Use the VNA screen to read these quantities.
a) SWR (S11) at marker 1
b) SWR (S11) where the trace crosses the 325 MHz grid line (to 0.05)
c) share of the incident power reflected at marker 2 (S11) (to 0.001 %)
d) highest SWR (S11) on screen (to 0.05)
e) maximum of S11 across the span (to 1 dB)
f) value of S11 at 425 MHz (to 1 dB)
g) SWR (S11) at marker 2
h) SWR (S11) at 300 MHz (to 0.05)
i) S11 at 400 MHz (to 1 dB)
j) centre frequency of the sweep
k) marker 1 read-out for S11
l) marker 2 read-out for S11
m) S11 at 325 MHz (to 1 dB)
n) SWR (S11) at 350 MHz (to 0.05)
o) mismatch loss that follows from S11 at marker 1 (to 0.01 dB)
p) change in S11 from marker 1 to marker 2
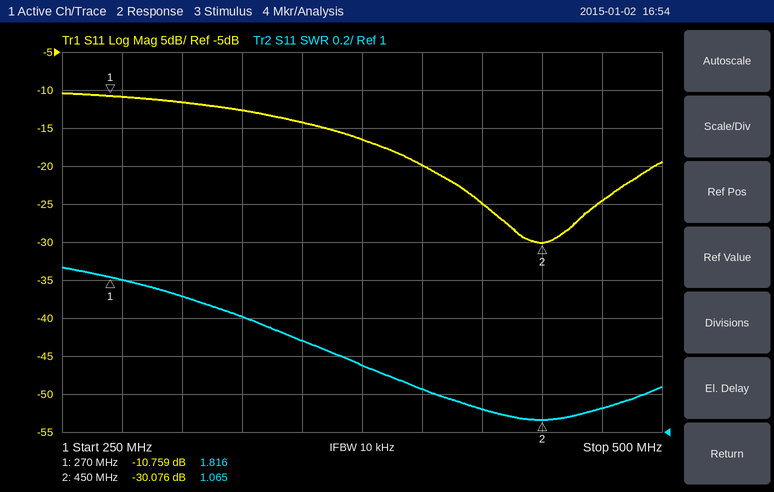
1.816
1.60
0.098 %
1.85
-10 dB
-25 dB
1.065
1.70
-20 dB
375 MHz
-10.759 dB
-30.076 dB
-13 dB
1.50
0.38 dB
-19.317 dB
